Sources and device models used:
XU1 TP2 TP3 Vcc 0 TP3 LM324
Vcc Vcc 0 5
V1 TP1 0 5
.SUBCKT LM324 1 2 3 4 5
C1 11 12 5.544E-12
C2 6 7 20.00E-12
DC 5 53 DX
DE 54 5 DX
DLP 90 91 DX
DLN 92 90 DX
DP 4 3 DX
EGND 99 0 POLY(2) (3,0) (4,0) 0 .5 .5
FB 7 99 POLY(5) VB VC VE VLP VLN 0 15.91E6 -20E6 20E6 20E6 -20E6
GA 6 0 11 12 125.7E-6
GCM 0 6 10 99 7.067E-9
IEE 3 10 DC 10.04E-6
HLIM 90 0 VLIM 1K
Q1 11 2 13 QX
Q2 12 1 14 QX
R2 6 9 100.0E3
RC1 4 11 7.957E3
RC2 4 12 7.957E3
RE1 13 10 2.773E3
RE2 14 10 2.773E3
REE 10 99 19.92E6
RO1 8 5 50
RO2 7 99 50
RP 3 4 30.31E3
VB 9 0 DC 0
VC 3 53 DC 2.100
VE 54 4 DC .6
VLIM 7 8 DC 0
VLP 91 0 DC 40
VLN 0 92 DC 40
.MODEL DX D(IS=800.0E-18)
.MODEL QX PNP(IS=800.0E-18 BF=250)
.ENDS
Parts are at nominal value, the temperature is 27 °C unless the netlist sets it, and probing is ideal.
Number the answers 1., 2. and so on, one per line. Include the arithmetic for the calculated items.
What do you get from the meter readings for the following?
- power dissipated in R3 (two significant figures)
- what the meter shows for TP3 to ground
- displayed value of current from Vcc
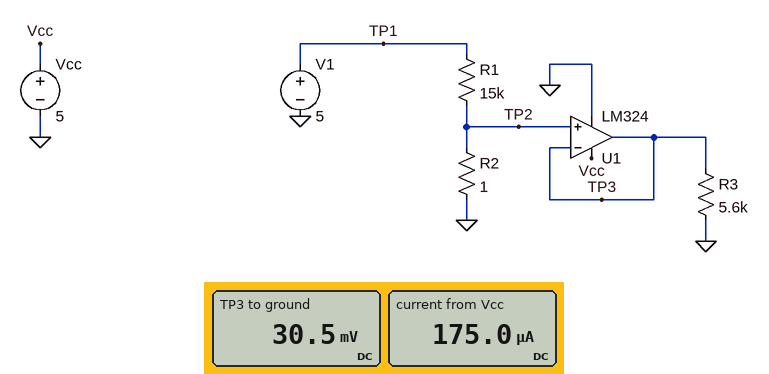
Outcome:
1. (30.5 mV)^2 / 5.6 kΩ = 170 nW
2. 30.5 mV
3. 175.0 µA
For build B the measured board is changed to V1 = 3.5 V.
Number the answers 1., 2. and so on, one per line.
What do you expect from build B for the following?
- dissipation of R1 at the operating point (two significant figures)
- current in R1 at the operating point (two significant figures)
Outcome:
1. 820 µW
2. 230 µA
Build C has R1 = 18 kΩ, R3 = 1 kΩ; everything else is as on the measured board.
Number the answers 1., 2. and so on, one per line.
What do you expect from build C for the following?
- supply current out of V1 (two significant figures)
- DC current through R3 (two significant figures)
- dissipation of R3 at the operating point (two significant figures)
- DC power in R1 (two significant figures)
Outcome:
1. 280 µA
2. 30 µA
3. 930 nW
4. 1.4 mW
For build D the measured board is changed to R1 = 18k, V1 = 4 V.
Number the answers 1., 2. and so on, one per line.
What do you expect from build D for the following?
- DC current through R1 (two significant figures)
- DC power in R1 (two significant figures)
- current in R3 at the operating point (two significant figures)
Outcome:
1. 220 µA
2. 890 µW
3. 5.4 µA
